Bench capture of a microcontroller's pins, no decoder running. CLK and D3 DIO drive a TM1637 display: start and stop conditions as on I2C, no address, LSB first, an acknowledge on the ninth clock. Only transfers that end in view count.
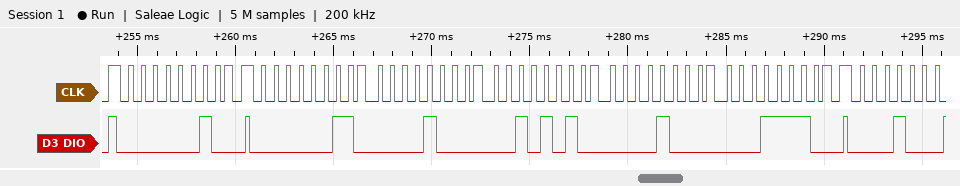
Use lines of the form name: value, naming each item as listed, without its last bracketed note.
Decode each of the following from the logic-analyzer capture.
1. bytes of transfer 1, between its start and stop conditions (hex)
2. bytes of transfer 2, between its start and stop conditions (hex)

bytes of transfer 1, between its start and stop conditions: 40
bytes of transfer 2, between its start and stop conditions: C0 10 54 10 78
